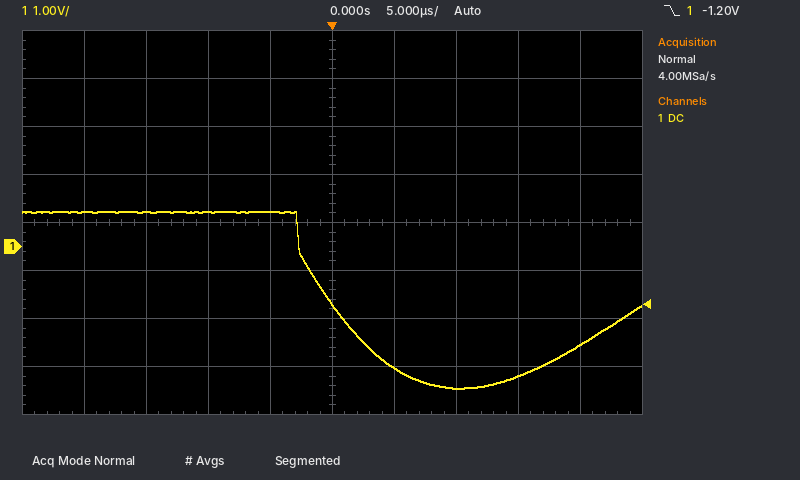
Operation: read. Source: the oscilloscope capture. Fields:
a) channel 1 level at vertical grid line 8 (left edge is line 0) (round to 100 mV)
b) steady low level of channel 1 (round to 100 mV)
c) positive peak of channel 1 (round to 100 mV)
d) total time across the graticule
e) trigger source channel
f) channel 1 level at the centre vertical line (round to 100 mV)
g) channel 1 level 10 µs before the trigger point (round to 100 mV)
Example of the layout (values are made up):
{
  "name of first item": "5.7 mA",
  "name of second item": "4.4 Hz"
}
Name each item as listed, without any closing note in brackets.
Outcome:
{
  "channel 1 level at vertical grid line 8 (left edge is line 0)": "-2.7 V",
  "steady low level of channel 1": "-2.9 V",
  "positive peak of channel 1": "700 mV",
  "total time across the graticule": "50 µs",
  "trigger source channel": "channel 1",
  "channel 1 level at the centre vertical line": "-1.2 V",
  "channel 1 level 10 µs before the trigger point": "700 mV"
}
